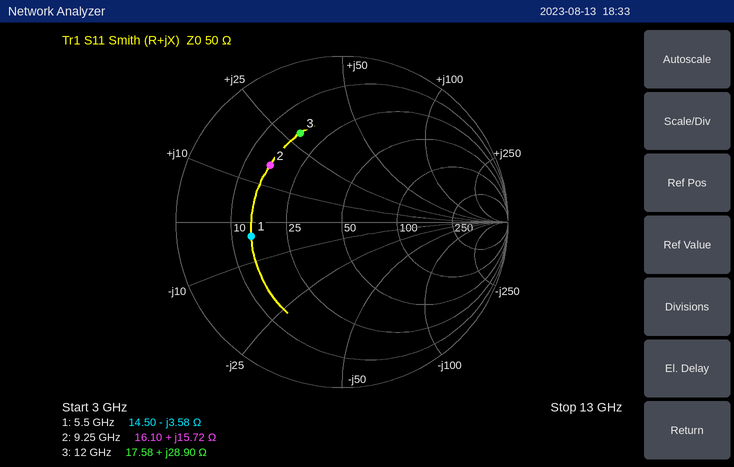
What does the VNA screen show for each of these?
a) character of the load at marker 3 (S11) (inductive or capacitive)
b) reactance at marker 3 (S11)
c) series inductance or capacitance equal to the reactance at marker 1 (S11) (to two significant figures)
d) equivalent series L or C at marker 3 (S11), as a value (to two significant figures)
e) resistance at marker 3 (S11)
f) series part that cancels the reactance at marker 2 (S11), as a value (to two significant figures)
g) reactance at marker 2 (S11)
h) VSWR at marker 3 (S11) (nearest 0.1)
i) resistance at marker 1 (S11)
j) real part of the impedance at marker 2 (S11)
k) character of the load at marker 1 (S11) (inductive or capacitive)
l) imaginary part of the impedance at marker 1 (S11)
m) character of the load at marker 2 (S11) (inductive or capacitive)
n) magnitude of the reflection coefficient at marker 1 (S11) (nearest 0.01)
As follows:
inductive
+28.90 Ω
8.1 pF
380 pH
17.58 Ω
1.1 pF
+15.72 Ω
3.9
14.50 Ω
16.10 Ω
capacitive
-3.58 Ω
inductive
0.55
